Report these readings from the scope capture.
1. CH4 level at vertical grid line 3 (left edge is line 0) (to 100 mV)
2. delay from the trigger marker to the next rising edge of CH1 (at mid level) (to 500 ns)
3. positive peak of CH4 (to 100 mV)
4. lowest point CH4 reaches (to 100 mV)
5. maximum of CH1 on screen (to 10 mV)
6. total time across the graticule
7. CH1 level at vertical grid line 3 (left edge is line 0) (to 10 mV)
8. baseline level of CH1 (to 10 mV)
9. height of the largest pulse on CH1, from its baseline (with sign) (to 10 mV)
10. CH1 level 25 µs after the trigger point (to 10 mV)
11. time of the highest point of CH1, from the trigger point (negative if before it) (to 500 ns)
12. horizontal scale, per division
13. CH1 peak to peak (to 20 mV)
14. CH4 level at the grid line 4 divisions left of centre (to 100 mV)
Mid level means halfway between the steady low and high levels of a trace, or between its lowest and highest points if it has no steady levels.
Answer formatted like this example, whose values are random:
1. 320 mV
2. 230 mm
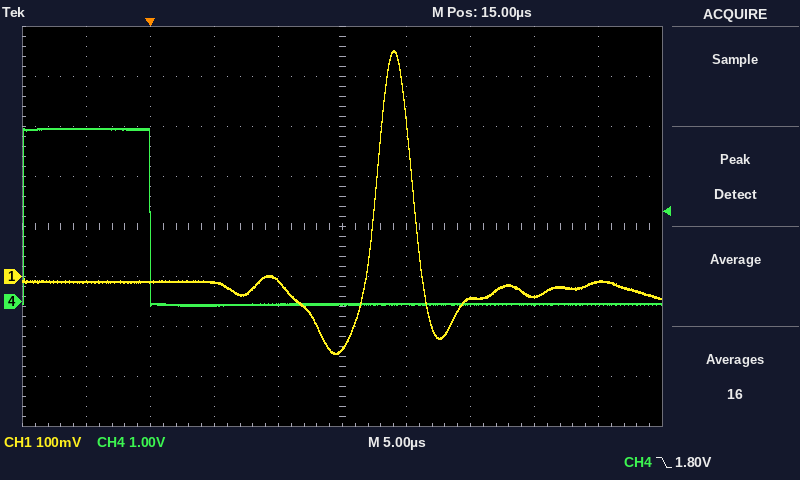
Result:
1. -100 mV
2. 17.5 µs
3. 3.5 V
4. -100 mV
5. 450 mV
6. 50 µs
7. -10 mV
8. -10 mV
9. +460 mV
10. -40 mV
11. +19.0 µs
12. 5 µs
13. 600 mV
14. 3.5 V
